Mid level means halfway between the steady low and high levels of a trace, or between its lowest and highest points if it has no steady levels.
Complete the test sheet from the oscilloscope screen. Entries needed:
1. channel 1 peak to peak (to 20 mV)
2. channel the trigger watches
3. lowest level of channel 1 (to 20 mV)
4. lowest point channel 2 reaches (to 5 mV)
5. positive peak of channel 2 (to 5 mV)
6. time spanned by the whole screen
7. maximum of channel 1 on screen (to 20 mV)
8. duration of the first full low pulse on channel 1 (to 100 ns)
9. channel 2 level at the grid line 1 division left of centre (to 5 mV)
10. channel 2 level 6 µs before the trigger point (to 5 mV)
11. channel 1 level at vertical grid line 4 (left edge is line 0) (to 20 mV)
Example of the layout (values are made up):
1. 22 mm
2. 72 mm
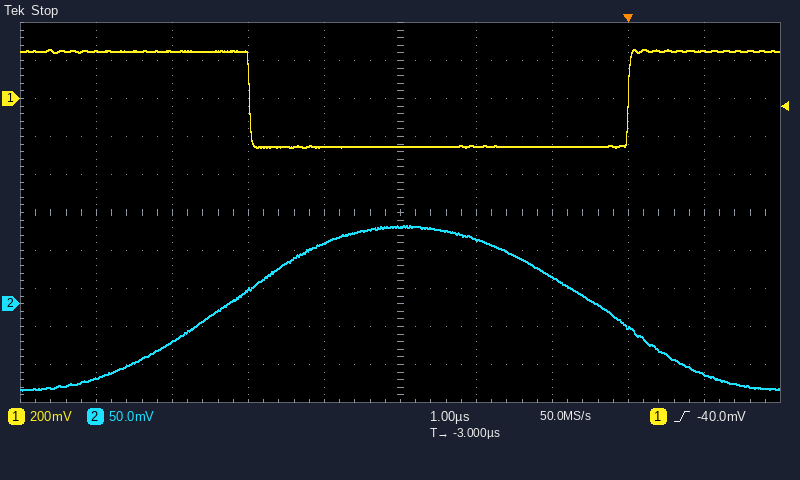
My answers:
1. 520 mV
2. channel 1
3. -260 mV
4. -115 mV
5. 105 mV
6. 10 µs
7. 260 mV
8. 5.0 µs
9. 80 mV
10. -50 mV
11. -260 mV
